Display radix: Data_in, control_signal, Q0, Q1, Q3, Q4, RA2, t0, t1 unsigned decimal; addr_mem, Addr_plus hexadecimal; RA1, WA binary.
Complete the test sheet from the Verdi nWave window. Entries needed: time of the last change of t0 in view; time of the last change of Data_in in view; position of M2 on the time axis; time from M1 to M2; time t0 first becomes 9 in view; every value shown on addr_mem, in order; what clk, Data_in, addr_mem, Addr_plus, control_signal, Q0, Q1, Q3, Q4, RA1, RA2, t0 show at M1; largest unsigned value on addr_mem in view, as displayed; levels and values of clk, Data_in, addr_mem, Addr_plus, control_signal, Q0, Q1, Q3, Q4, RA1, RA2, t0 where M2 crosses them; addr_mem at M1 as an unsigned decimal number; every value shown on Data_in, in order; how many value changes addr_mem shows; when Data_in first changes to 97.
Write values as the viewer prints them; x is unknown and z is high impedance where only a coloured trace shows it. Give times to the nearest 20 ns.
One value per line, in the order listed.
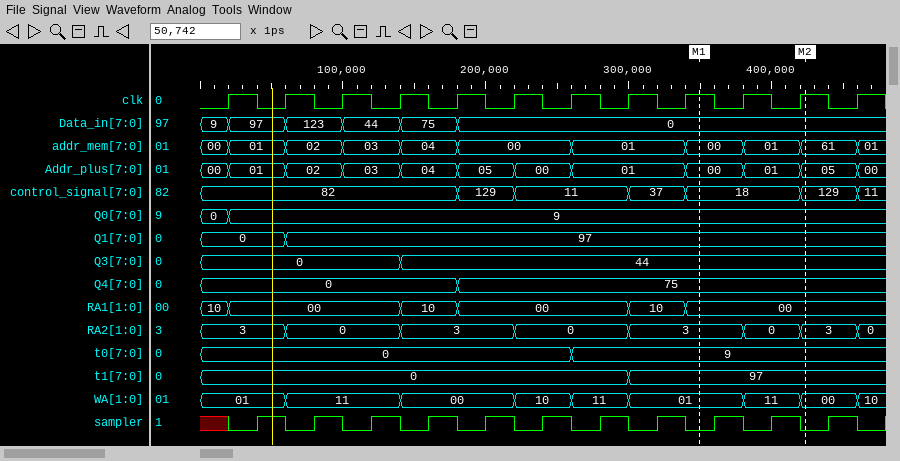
260 ns
180 ns
420 ns
80 ns
260 ns
00, 01, 02, 03, 04, 00, 01, 00, 01, 61, 01
clk=1, Data_in=0, addr_mem=00, Addr_plus=00, control_signal=18, Q0=9, Q1=97, Q3=44, Q4=75, RA1=00, RA2=3, t0=9
61
clk=1, Data_in=0, addr_mem=61, Addr_plus=05, control_signal=129, Q0=9, Q1=97, Q3=44, Q4=75, RA1=00, RA2=3, t0=9
0
9, 97, 123, 44, 75, 0
10
20 ns
